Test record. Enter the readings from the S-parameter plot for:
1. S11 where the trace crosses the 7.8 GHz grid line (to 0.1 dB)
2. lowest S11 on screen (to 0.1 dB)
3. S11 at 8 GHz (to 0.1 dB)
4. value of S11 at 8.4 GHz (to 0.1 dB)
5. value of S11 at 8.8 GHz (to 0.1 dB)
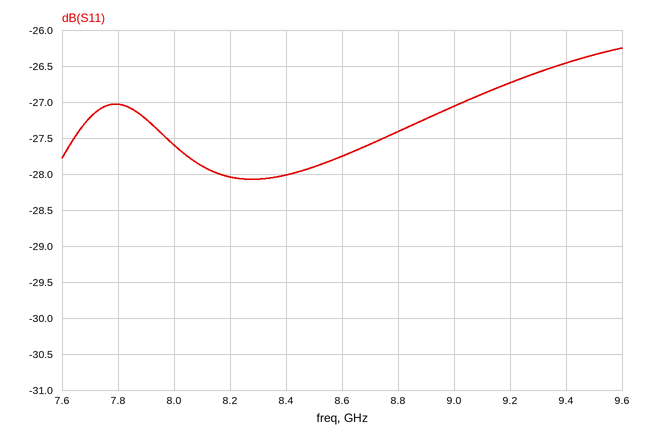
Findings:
-27.0 dB
-28.1 dB
-27.6 dB
-28.0 dB
-27.4 dB
